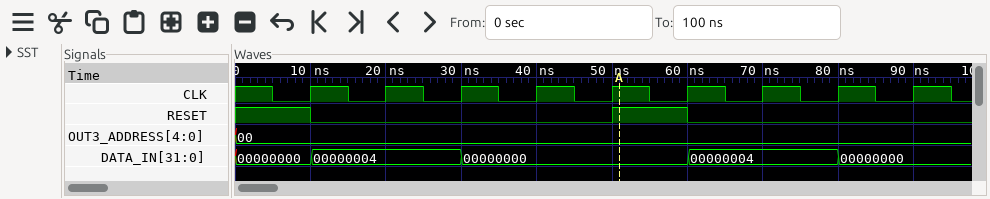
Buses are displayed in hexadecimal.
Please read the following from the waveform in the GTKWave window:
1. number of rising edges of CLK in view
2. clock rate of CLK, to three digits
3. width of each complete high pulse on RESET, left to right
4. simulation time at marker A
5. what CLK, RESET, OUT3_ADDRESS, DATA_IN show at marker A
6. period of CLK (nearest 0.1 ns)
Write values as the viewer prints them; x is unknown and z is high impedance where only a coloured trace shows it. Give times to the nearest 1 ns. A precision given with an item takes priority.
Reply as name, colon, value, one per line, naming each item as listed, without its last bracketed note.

number of rising edges of CLK in view: 9
clock rate of CLK, to three digits: 100 MHz
width of each complete high pulse on RESET, left to right: 10 ns
simulation time at marker A: 51 ns
what CLK, RESET, OUT3_ADDRESS, DATA_IN show at marker A: CLK=1, RESET=1, OUT3_ADDRESS=00, DATA_IN=00000000
period of CLK: 10 ns
